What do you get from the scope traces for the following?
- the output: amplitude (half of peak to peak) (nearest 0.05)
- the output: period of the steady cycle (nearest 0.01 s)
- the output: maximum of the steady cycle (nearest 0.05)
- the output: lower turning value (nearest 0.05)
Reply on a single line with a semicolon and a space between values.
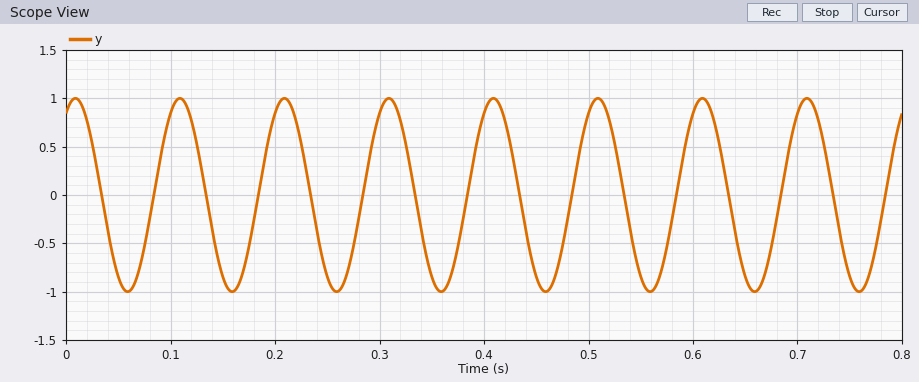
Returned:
1.00; 0.10 s; 1.00; -1.00
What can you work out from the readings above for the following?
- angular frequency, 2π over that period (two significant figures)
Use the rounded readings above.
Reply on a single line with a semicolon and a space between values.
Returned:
63 rad/s
